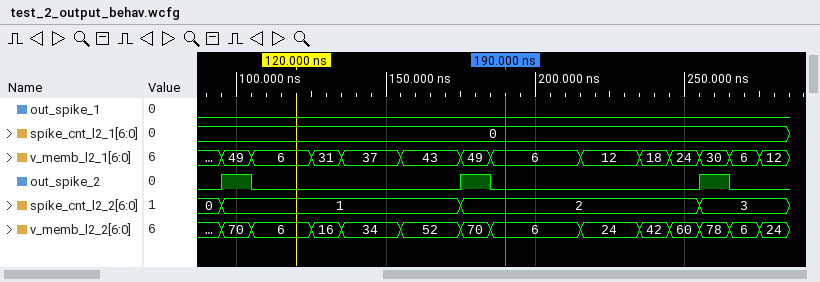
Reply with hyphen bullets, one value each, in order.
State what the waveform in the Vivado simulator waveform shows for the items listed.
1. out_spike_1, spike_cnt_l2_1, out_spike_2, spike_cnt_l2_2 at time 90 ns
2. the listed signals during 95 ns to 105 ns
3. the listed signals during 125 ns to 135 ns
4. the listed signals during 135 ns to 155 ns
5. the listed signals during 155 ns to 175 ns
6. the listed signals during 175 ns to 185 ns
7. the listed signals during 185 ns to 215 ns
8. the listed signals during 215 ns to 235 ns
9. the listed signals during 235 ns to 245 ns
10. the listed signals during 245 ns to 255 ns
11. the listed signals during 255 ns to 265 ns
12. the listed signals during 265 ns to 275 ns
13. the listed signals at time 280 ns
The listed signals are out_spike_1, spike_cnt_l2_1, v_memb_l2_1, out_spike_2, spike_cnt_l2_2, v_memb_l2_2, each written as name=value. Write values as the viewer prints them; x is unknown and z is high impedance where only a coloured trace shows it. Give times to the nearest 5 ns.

- out_spike_1=0, spike_cnt_l2_1=0, out_spike_2=0, spike_cnt_l2_2=0
- out_spike_1=0, spike_cnt_l2_1=0, v_memb_l2_1=49, out_spike_2=1, spike_cnt_l2_2=1, v_memb_l2_2=70
- out_spike_1=0, spike_cnt_l2_1=0, v_memb_l2_1=31, out_spike_2=0, spike_cnt_l2_2=1, v_memb_l2_2=16
- out_spike_1=0, spike_cnt_l2_1=0, v_memb_l2_1=37, out_spike_2=0, spike_cnt_l2_2=1, v_memb_l2_2=34
- out_spike_1=0, spike_cnt_l2_1=0, v_memb_l2_1=43, out_spike_2=0, spike_cnt_l2_2=1, v_memb_l2_2=52
- out_spike_1=0, spike_cnt_l2_1=0, v_memb_l2_1=49, out_spike_2=1, spike_cnt_l2_2=2, v_memb_l2_2=70
- out_spike_1=0, spike_cnt_l2_1=0, v_memb_l2_1=6, out_spike_2=0, spike_cnt_l2_2=2, v_memb_l2_2=6
- out_spike_1=0, spike_cnt_l2_1=0, v_memb_l2_1=12, out_spike_2=0, spike_cnt_l2_2=2, v_memb_l2_2=24
- out_spike_1=0, spike_cnt_l2_1=0, v_memb_l2_1=18, out_spike_2=0, spike_cnt_l2_2=2, v_memb_l2_2=42
- out_spike_1=0, spike_cnt_l2_1=0, v_memb_l2_1=24, out_spike_2=0, spike_cnt_l2_2=2, v_memb_l2_2=60
- out_spike_1=0, spike_cnt_l2_1=0, v_memb_l2_1=30, out_spike_2=1, spike_cnt_l2_2=3, v_memb_l2_2=78
- out_spike_1=0, spike_cnt_l2_1=0, v_memb_l2_1=6, out_spike_2=0, spike_cnt_l2_2=3, v_memb_l2_2=6
- out_spike_1=0, spike_cnt_l2_1=0, v_memb_l2_1=12, out_spike_2=0, spike_cnt_l2_2=3, v_memb_l2_2=24
